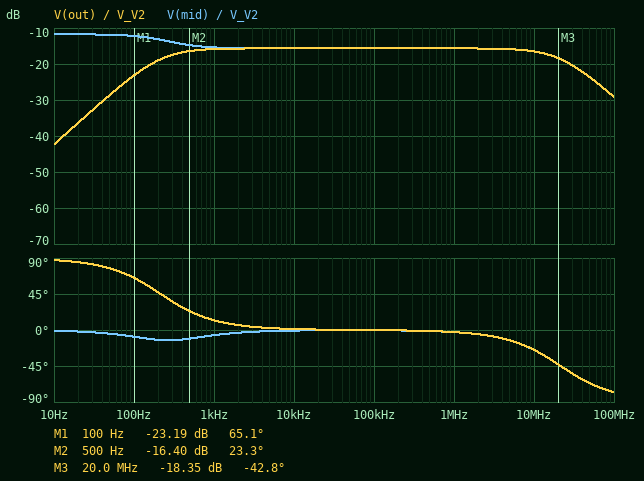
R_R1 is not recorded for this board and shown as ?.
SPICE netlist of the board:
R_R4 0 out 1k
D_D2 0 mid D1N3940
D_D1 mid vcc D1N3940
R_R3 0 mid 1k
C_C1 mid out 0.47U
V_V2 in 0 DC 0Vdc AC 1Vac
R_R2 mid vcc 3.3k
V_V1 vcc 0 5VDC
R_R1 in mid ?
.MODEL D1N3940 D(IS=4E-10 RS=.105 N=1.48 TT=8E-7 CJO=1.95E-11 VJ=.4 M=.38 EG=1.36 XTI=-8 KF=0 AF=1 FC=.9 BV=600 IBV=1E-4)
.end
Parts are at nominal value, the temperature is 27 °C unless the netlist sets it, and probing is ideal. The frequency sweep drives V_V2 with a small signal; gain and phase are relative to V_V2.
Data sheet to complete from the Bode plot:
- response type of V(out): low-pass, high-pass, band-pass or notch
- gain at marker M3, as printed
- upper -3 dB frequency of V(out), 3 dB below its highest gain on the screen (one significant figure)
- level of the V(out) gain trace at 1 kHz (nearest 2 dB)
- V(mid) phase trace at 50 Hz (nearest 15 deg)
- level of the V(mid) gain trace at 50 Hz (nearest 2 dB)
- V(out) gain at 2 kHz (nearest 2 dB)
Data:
band-pass
-18.35 dB
20 MHz
-16 dB
0 deg
-12 dB
-16 dB
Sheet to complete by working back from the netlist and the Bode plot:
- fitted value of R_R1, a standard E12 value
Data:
2.2 kΩ
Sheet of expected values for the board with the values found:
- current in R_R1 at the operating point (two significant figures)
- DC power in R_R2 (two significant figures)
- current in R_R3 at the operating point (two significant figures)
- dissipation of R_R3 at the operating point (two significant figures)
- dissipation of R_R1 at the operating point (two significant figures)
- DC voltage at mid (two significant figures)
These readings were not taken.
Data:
390 µA
5.2 mW
860 µA
740 µW
340 µW
860 mV
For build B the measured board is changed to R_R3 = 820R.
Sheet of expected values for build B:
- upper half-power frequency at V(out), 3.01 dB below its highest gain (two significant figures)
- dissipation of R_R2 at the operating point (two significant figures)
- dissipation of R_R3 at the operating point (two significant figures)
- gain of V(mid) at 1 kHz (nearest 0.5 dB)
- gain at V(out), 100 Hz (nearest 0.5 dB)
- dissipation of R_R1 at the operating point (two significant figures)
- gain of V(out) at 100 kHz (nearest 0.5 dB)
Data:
23 MHz
5.4 mW
720 µW
-16.0 dB
-24.0 dB
270 µW
-16.5 dB
